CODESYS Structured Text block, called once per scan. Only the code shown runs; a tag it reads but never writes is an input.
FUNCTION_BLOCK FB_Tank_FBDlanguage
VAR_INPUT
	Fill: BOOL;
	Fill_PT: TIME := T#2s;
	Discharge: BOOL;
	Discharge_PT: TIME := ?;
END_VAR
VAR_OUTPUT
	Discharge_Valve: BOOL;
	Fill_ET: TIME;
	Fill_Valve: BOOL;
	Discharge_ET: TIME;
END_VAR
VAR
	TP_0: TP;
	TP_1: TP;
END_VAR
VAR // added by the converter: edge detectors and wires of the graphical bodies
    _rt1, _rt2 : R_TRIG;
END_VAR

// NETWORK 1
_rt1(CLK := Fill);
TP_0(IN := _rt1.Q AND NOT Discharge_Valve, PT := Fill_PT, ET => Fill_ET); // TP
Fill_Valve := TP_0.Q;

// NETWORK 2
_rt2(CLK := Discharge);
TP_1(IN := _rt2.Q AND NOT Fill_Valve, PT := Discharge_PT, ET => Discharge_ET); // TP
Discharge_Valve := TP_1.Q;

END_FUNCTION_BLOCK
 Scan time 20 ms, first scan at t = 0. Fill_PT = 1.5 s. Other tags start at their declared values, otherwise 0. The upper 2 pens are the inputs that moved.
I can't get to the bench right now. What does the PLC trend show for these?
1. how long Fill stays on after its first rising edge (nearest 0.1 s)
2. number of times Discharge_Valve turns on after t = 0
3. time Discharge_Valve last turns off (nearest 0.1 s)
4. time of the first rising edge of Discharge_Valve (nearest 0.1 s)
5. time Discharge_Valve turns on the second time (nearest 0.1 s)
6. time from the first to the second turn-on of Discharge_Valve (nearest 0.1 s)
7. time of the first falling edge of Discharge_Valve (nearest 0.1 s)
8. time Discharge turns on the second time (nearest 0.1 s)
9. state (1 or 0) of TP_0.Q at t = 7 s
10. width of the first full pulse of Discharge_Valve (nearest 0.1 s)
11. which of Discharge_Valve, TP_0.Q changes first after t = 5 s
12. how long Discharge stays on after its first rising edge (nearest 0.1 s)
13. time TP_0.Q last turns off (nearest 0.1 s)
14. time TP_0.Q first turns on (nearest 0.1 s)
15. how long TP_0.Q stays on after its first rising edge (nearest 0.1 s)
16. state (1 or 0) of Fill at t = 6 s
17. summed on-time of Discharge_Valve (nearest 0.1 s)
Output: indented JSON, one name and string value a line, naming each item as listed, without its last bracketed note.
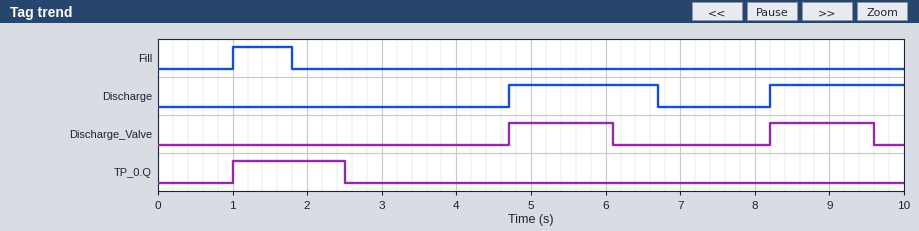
{
  "how long Fill stays on after its first rising edge": "0.8 s",
  "number of times Discharge_Valve turns on after t = 0": "2",
  "time Discharge_Valve last turns off": "9.6 s",
  "time of the first rising edge of Discharge_Valve": "4.7 s",
  "time Discharge_Valve turns on the second time": "8.2 s",
  "time from the first to the second turn-on of Discharge_Valve": "3.5 s",
  "time of the first falling edge of Discharge_Valve": "6.1 s",
  "time Discharge turns on the second time": "8.2 s",
  "state (1 or 0) of TP_0.Q at t = 7 s": "0",
  "width of the first full pulse of Discharge_Valve": "1.4 s",
  "which of Discharge_Valve, TP_0.Q changes first after t = 5 s": "Discharge_Valve",
  "how long Discharge stays on after its first rising edge": "2.0 s",
  "time TP_0.Q last turns off": "2.5 s",
  "time TP_0.Q first turns on": "1.0 s",
  "how long TP_0.Q stays on after its first rising edge": "1.5 s",
  "state (1 or 0) of Fill at t = 6 s": "0",
  "summed on-time of Discharge_Valve": "2.8 s"
}
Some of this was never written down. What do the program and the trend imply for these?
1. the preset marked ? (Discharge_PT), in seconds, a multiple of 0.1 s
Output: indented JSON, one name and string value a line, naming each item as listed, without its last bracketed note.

{
  "the preset marked ? (Discharge_PT), in seconds, a multiple of 0.1 s": "1.4 s"
}
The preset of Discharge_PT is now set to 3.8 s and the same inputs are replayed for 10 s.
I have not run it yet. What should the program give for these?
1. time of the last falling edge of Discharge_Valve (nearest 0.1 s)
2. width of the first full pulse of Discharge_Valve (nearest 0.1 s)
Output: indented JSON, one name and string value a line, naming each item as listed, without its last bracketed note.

{
  "time of the last falling edge of Discharge_Valve": "8.5 s",
  "width of the first full pulse of Discharge_Valve": "3.8 s"
}
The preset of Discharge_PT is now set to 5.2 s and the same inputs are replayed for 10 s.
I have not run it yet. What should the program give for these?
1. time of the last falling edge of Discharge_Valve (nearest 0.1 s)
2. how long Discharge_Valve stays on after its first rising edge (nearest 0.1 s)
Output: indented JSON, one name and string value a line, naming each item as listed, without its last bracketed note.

{
  "time of the last falling edge of Discharge_Valve": "9.9 s",
  "how long Discharge_Valve stays on after its first rising edge": "5.2 s"
}
